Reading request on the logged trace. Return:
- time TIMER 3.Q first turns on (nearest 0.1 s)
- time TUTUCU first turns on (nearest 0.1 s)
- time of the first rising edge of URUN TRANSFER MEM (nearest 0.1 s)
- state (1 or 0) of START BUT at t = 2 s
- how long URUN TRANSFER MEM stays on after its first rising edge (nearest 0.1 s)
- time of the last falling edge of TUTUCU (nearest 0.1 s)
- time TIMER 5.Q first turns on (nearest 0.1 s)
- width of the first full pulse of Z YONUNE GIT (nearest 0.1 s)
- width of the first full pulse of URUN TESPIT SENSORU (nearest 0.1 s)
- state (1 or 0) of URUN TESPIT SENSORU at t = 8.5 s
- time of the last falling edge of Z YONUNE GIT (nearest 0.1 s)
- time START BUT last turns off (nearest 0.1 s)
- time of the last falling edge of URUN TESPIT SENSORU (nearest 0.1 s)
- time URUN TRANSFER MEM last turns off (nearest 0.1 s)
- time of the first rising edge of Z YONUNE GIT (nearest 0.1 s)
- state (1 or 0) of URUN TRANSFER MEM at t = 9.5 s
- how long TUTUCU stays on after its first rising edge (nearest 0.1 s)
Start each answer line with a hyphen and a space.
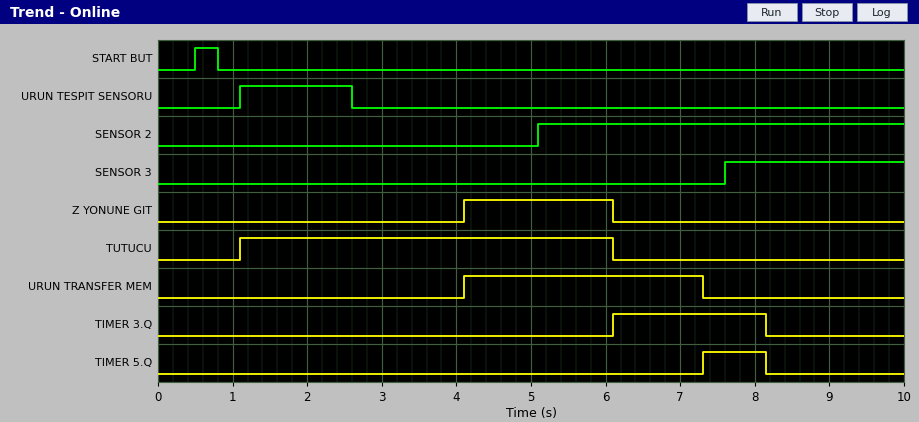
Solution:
- 6.1 s
- 1.1 s
- 4.1 s
- 0
- 3.2 s
- 6.1 s
- 7.3 s
- 2.0 s
- 1.5 s
- 0
- 6.1 s
- 0.8 s
- 2.6 s
- 7.3 s
- 4.1 s
- 0
- 5.0 s
